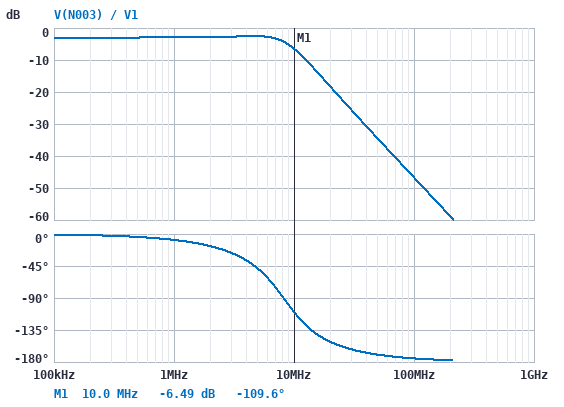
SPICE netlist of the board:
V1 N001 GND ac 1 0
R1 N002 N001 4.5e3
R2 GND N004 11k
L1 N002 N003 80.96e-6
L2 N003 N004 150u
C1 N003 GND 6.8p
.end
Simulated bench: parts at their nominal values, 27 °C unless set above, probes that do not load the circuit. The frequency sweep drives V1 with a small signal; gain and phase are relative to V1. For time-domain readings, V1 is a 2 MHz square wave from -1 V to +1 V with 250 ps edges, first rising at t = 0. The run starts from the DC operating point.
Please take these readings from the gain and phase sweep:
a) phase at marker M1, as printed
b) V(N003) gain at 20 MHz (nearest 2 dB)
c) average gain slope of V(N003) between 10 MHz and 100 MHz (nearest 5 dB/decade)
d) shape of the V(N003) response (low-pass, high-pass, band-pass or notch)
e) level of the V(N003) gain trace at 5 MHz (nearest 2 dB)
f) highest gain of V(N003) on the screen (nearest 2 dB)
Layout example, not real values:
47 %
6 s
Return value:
-109.6 deg
-18 dB
-40 dB/decade
low-pass
-2 dB
-2 dB
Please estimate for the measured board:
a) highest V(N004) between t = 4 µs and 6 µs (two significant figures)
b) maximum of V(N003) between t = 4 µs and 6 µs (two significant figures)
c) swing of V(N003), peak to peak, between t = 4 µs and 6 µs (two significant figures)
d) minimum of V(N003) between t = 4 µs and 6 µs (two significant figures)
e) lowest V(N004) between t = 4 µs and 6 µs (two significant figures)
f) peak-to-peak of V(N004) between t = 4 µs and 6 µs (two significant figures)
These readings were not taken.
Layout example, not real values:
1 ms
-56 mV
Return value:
810 mV
860 mV
1.7 V
-860 mV
-810 mV
1.6 V
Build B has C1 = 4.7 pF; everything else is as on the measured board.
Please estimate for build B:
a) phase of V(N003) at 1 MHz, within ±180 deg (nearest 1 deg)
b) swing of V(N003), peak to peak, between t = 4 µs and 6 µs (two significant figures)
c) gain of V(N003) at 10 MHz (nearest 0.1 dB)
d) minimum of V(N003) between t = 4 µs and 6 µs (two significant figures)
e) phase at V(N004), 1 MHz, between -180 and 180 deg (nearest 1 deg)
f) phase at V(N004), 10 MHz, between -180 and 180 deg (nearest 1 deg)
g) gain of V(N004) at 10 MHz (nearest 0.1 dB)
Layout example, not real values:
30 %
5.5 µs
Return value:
-6 deg
1.9 V
-2.9 dB
-950 mV
-11 deg
-132 deg
-5.3 dB
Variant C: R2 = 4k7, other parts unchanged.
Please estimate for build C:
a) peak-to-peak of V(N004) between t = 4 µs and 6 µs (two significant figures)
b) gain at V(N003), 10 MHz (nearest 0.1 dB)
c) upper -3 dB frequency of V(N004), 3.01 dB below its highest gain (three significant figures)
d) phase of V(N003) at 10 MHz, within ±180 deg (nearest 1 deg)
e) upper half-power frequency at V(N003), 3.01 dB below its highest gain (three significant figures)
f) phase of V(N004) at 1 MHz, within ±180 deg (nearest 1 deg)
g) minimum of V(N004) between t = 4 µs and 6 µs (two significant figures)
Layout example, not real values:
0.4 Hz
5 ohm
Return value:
1.2 V
-5.3 dB
8.32 MHz
-107 deg
10.0 MHz
-15 deg
-600 mV
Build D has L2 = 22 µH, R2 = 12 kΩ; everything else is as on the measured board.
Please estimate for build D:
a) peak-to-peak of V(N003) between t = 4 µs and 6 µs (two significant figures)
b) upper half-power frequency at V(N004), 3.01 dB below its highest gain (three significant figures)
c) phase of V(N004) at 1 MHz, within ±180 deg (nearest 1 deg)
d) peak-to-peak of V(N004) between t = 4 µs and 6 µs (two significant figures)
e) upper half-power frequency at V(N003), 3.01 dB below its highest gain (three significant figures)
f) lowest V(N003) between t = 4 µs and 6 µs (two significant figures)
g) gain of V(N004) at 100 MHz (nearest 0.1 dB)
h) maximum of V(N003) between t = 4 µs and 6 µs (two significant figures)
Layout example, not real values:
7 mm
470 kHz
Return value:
1.6 V
8.37 MHz
-10 deg
1.6 V
8.40 MHz
-810 mV
-50.3 dB
810 mV
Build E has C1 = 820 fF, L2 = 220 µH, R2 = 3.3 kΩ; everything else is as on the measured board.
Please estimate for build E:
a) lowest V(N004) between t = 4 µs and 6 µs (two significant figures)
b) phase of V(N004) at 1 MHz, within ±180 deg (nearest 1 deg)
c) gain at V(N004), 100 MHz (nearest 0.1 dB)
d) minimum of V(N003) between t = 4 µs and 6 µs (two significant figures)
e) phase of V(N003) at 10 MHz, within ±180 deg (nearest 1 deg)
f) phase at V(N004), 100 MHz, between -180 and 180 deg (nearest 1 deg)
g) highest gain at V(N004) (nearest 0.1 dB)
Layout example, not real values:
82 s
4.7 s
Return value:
-420 mV
-14 deg
-60.4 dB
-1.7 V
0 deg
97 deg
-7.5 dB
